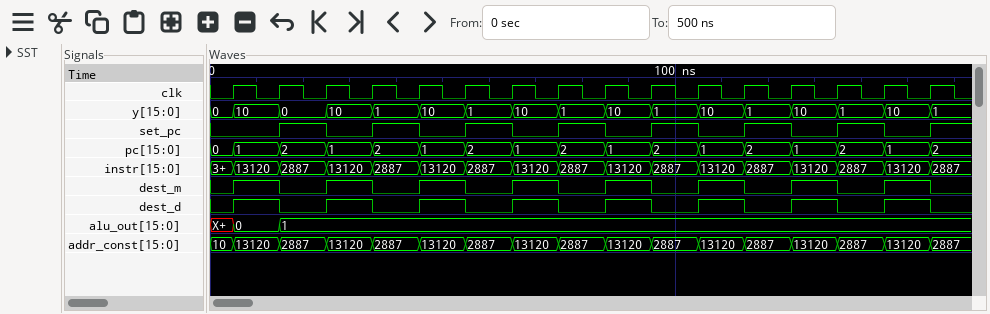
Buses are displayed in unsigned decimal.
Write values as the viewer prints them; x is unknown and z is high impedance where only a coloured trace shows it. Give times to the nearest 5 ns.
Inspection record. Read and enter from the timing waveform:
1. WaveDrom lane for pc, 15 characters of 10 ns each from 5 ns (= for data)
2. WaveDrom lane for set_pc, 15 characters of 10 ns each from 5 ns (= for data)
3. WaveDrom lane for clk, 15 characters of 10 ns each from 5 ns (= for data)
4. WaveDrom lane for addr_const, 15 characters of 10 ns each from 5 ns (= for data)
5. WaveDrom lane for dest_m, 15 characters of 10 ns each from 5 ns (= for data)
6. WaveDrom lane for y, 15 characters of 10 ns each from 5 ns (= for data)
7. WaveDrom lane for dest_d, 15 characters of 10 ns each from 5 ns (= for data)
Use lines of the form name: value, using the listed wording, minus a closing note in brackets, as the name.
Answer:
WaveDrom lane for pc, 15 characters of 10 ns each from 5 ns: {name: 'pc', wave: '===============', data: '1 2 1 2 1 2 1 2 1 2 1 2 1 2 1'}
WaveDrom lane for set_pc, 15 characters of 10 ns each from 5 ns: {name: 'set_pc', wave: '010101010101010'}
WaveDrom lane for clk, 15 characters of 10 ns each from 5 ns: {name: 'clk', wave: 'p..............'}
WaveDrom lane for addr_const, 15 characters of 10 ns each from 5 ns: {name: 'addr_const', wave: '===============', data: '13120 2887 13120 2887 13120 2887 13120 2887 13120 2887 13120 2887 13120 2887 13120'}
WaveDrom lane for dest_m, 15 characters of 10 ns each from 5 ns: {name: 'dest_m', wave: '101010101010101'}
WaveDrom lane for y, 15 characters of 10 ns each from 5 ns: {name: 'y', wave: '===============', data: '10 0 10 1 10 1 10 1 10 1 10 1 10 1 10'}
WaveDrom lane for dest_d, 15 characters of 10 ns each from 5 ns: {name: 'dest_d', wave: '101010101010101'}
